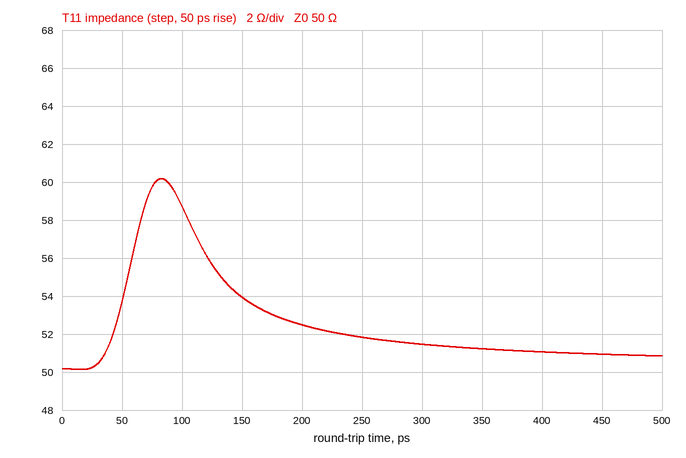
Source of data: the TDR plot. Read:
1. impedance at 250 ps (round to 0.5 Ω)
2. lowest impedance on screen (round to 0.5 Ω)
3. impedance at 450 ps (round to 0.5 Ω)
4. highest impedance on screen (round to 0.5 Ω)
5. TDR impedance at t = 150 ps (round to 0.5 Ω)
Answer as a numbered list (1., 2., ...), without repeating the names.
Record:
1. 52.0 Ω
2. 50.0 Ω
3. 51.0 Ω
4. 60.0 Ω
5. 54.0 Ω
